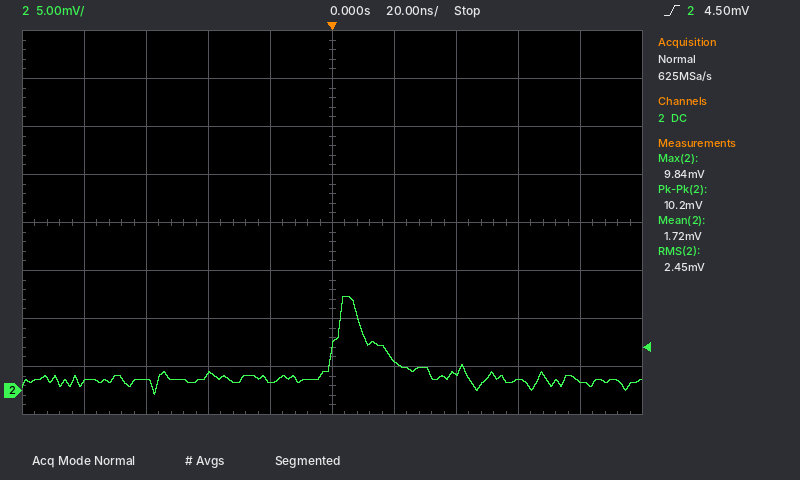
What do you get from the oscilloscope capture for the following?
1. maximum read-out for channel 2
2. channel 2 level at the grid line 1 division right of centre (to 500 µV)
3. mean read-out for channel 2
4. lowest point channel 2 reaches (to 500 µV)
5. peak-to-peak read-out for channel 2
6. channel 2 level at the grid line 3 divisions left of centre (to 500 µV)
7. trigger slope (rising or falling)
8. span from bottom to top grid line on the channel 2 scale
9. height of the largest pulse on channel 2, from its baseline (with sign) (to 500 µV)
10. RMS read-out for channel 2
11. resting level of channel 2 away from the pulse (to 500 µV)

9.84 mV
3.0 mV
1.72 mV
-500 µV
10.2 mV
1.0 mV
rising
40 mV
+8.5 mV
2.45 mV
1.0 mV
